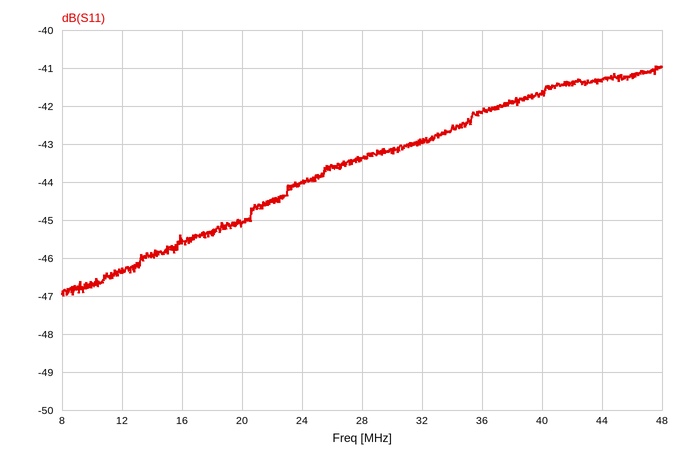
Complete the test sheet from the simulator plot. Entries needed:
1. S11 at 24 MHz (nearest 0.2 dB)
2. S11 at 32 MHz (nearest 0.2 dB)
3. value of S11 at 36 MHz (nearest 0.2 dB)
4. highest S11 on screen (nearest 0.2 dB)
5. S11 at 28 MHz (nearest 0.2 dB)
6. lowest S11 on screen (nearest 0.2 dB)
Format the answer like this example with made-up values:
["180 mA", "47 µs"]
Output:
["-44.0 dB", "-43.0 dB", "-42.2 dB", "-41.0 dB", "-43.4 dB", "-47.0 dB"]
